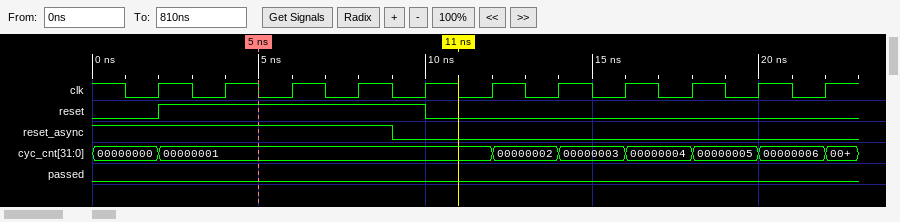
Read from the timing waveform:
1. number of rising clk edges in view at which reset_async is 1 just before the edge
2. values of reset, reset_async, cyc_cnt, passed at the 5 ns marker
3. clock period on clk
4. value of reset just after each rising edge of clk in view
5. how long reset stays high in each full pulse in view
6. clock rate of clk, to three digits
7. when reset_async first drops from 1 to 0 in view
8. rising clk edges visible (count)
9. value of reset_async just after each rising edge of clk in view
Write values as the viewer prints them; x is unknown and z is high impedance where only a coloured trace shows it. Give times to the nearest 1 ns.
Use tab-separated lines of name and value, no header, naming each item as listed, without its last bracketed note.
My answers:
number of rising clk edges in view at which reset_async is 1 just before the edge	4
values of reset, reset_async, cyc_cnt, passed at the 5 ns marker	reset=1, reset_async=1, cyc_cnt=00000001, passed=0
clock period on clk	2 ns
value of reset just after each rising edge of clk in view	1 1 1 1 0 0 0 0 0 0 0
how long reset stays high in each full pulse in view	8 ns
clock rate of clk, to three digits	500 MHz
when reset_async first drops from 1 to 0 in view	9 ns
rising clk edges visible	11
value of reset_async just after each rising edge of clk in view	1 1 1 1 0 0 0 0 0 0 0
